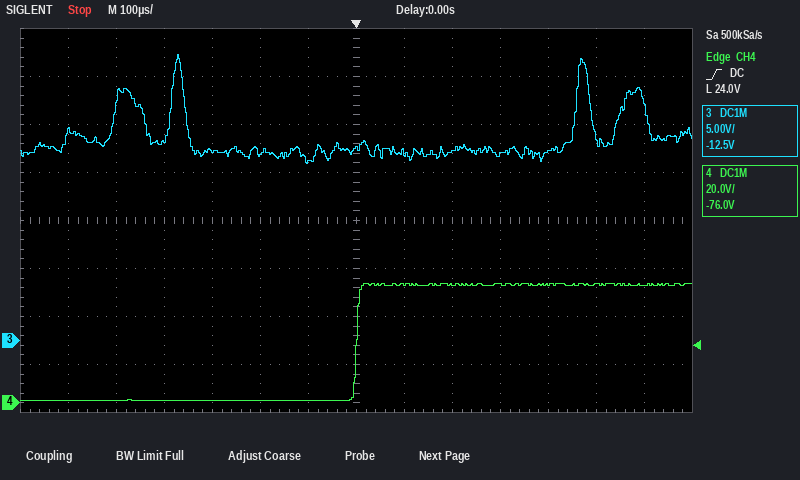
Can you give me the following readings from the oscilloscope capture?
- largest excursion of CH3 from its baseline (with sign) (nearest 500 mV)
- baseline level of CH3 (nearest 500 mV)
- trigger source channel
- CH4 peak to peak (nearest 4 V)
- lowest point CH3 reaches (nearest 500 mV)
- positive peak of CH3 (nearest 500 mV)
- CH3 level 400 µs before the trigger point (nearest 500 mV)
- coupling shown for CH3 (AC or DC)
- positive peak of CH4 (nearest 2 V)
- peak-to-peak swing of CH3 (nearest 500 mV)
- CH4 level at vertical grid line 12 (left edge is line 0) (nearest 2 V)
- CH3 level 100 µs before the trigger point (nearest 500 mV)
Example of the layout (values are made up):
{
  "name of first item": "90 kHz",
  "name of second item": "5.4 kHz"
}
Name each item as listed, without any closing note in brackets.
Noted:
{
  "largest excursion of CH3 from its baseline (with sign)": "+10.0 V",
  "baseline level of CH3": "20.0 V",
  "trigger source channel": "CH4",
  "CH4 peak to peak": "48 V",
  "lowest point CH3 reaches": "18.5 V",
  "positive peak of CH3": "30.0 V",
  "CH3 level 400 µs before the trigger point": "21.0 V",
  "coupling shown for CH3": "DC",
  "positive peak of CH4": "50 V",
  "peak-to-peak swing of CH3": "11.5 V",
  "CH4 level at vertical grid line 12 (left edge is line 0)": "50 V",
  "CH3 level 100 µs before the trigger point": "18.5 V"
}
